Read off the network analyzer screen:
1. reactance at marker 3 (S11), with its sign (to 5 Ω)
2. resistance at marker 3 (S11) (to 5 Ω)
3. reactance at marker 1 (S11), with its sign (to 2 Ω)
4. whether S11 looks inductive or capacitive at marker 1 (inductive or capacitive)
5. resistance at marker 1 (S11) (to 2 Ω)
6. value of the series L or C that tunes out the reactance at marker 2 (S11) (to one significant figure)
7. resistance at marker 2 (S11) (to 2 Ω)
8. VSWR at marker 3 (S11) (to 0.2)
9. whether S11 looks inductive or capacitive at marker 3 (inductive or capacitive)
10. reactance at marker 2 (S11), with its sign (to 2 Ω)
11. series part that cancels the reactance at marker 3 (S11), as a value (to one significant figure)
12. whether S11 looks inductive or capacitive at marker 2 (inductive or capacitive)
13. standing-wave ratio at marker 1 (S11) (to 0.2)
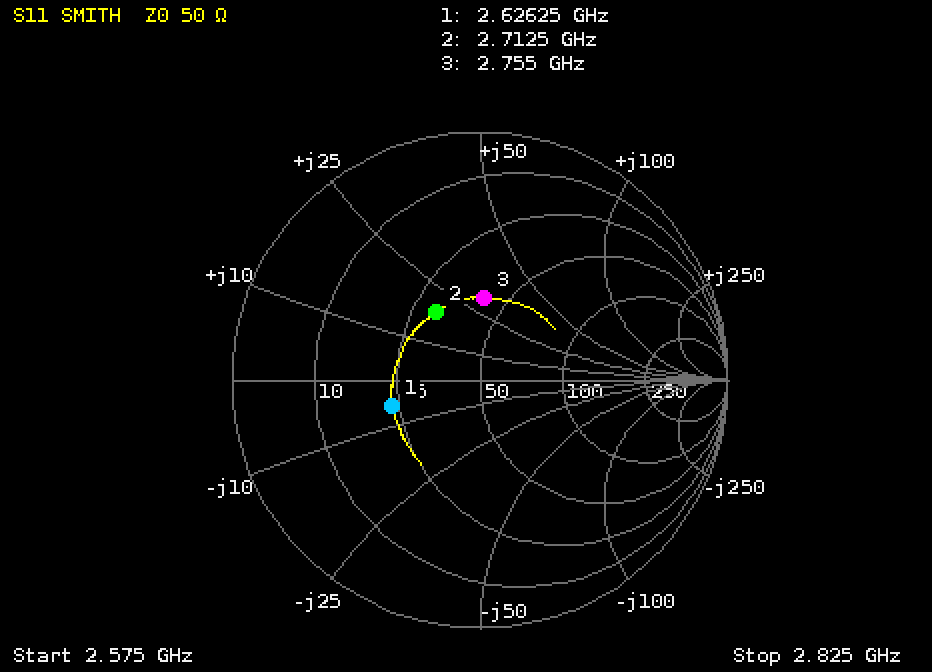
+30 Ω
40 Ω
-6 Ω
capacitive
24 Ω
3 pF
30 Ω
2.0
inductive
+18 Ω
2 pF
inductive
2.2
